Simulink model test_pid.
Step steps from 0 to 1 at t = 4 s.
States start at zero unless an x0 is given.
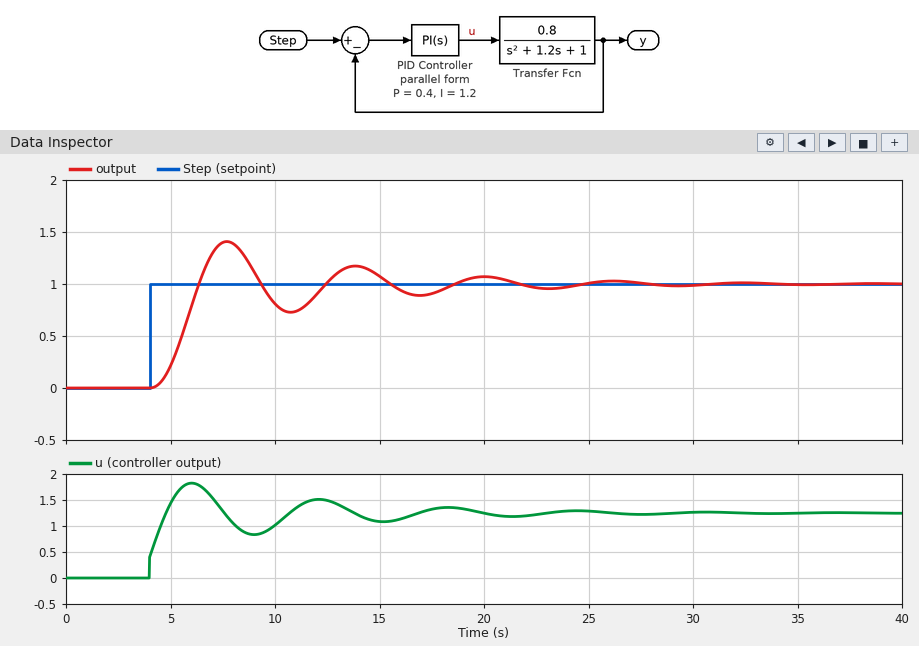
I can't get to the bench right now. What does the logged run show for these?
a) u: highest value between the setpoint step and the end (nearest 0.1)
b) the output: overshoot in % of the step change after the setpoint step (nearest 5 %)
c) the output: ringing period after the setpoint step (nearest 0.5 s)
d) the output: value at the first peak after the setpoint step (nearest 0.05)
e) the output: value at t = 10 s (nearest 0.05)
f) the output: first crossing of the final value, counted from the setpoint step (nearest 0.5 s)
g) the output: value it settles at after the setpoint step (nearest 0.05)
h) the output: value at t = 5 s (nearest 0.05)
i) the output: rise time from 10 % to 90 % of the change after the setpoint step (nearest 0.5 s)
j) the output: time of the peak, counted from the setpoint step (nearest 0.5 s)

1.8
40 %
6.0 s
1.40
0.80
2.5 s
1.00
0.20
1.5 s
3.5 s
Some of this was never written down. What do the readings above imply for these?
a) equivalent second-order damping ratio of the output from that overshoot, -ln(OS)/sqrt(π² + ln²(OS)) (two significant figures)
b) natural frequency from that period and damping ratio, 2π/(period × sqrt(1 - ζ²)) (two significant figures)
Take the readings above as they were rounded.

0.28
1.1 rad/s
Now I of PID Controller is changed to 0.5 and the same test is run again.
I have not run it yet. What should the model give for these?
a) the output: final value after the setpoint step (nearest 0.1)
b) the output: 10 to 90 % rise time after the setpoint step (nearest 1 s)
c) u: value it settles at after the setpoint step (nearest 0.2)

1.0
3 s
1.2
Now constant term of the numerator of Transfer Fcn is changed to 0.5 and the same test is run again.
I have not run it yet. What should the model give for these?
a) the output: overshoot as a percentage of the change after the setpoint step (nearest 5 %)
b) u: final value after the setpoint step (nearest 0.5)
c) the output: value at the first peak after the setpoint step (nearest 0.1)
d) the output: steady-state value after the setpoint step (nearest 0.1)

20 %
2.0
1.2
1.0
